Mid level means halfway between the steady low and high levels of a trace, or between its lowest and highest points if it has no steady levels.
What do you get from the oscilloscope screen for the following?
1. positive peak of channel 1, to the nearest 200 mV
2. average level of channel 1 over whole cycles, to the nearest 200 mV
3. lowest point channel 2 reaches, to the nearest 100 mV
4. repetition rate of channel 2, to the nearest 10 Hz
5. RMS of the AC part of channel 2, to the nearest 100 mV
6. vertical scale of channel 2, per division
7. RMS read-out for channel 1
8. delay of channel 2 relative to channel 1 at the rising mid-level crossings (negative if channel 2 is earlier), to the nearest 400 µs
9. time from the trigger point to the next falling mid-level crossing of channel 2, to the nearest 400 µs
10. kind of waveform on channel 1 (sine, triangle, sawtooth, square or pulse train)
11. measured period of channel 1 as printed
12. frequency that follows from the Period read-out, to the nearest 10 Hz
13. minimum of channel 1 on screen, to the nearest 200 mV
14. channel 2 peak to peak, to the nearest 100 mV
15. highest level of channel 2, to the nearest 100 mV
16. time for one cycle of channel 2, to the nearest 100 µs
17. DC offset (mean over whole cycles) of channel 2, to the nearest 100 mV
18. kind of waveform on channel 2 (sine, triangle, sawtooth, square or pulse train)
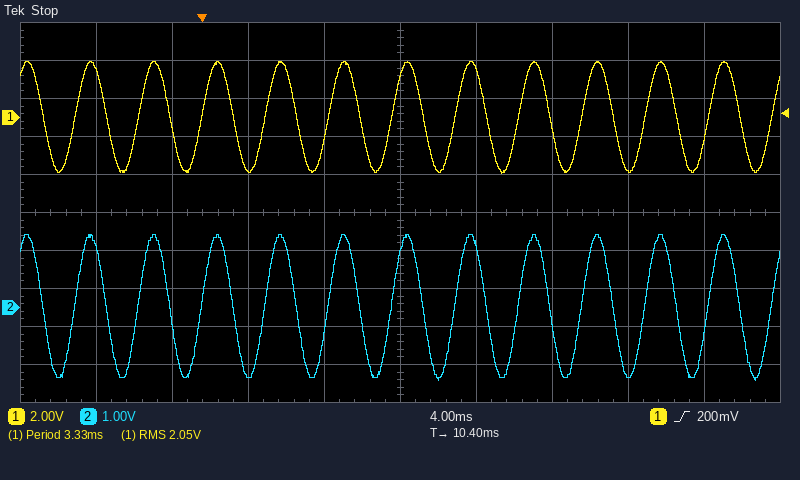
3.0 V
0.0 V
-1.9 V
300 Hz
1.3 V
1 V
2.05 V
0.0 ms
1.6 ms
sine
3.33 ms
300 Hz
-3.0 V
3.8 V
1.9 V
3.3 ms
0.0 V
sine
